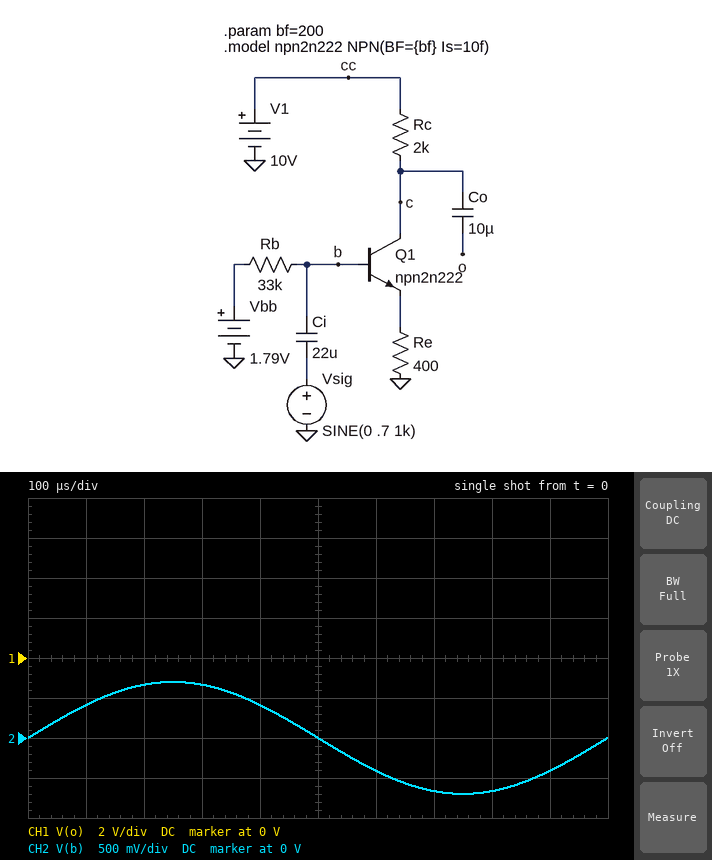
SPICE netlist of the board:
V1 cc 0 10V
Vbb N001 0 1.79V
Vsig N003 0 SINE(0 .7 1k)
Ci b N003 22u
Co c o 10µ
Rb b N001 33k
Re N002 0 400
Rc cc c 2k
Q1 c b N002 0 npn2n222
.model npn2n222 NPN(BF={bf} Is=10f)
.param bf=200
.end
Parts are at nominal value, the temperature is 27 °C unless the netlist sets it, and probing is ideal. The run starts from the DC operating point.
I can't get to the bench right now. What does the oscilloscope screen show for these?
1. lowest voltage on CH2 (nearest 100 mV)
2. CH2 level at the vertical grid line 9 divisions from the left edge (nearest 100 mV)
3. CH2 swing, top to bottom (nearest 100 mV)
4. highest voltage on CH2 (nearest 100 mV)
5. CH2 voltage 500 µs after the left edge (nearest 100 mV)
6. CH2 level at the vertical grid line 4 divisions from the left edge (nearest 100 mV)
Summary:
-700 mV
-400 mV
1.4 V
700 mV
0 V
400 mV
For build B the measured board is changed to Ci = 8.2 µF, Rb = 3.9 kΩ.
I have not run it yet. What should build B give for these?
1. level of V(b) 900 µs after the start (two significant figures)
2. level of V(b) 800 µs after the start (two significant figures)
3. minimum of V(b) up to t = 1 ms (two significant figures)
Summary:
-360 mV
-620 mV
-660 mV
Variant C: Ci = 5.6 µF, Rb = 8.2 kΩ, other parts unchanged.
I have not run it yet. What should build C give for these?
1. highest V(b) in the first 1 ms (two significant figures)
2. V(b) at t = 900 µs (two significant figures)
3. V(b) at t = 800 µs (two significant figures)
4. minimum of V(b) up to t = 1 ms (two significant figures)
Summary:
710 mV
-380 mV
-640 mV
-670 mV
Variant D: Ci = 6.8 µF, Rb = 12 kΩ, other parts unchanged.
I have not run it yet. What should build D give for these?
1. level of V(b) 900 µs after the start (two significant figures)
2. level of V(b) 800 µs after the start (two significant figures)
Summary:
-390 mV
-650 mV
